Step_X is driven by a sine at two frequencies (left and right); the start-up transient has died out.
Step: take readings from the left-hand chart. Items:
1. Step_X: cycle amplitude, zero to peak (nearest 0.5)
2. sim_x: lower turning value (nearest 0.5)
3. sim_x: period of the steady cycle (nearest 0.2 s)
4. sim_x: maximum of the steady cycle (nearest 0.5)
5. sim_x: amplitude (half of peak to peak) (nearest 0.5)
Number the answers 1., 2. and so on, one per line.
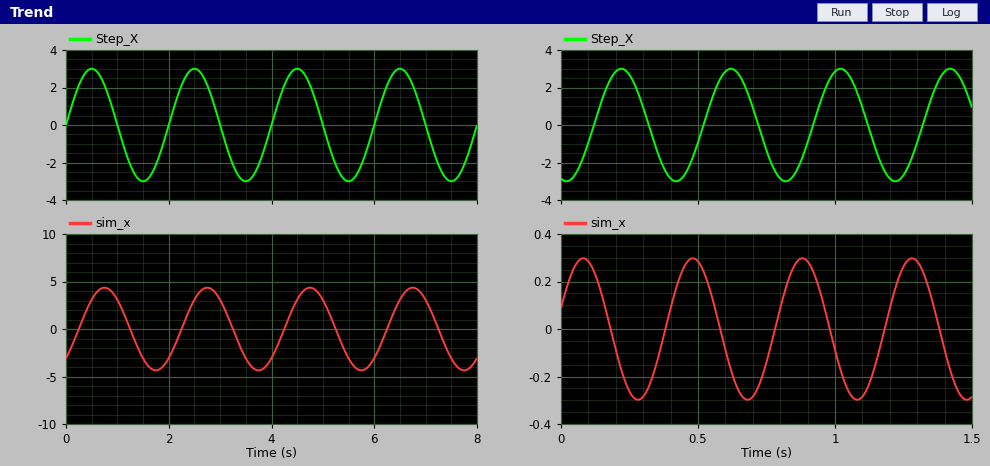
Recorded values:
1. 3.0
2. -4.5
3. 2.0 s
4. 4.5
5. 4.5
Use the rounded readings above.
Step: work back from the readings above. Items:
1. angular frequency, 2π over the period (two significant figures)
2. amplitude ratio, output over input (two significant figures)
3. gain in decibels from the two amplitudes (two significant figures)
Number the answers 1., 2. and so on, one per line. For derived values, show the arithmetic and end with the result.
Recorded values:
1. 2π / 2 = 3.1 rad/s
2. 4.5 / 3 = 1.5
3. 20 log10(4.5 / 3) = 3.5 dB
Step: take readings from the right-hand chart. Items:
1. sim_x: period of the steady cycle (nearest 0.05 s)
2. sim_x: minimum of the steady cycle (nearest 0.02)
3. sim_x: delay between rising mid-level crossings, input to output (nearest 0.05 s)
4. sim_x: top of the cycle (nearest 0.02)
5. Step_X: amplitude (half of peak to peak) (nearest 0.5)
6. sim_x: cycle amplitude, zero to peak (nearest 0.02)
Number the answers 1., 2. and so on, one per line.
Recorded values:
1. 0.40 s
2. -0.30
3. 0.25 s
4. 0.30
5. 3.0
6. 0.30
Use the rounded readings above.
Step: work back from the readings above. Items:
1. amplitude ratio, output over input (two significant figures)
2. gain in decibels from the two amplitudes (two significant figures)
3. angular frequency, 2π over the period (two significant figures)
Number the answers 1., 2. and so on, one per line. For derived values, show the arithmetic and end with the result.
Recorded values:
1. 0.3 / 3 = 0.10
2. 20 log10(0.3 / 3) = -20 dB
3. 2π / 0.4 = 16 rad/s
